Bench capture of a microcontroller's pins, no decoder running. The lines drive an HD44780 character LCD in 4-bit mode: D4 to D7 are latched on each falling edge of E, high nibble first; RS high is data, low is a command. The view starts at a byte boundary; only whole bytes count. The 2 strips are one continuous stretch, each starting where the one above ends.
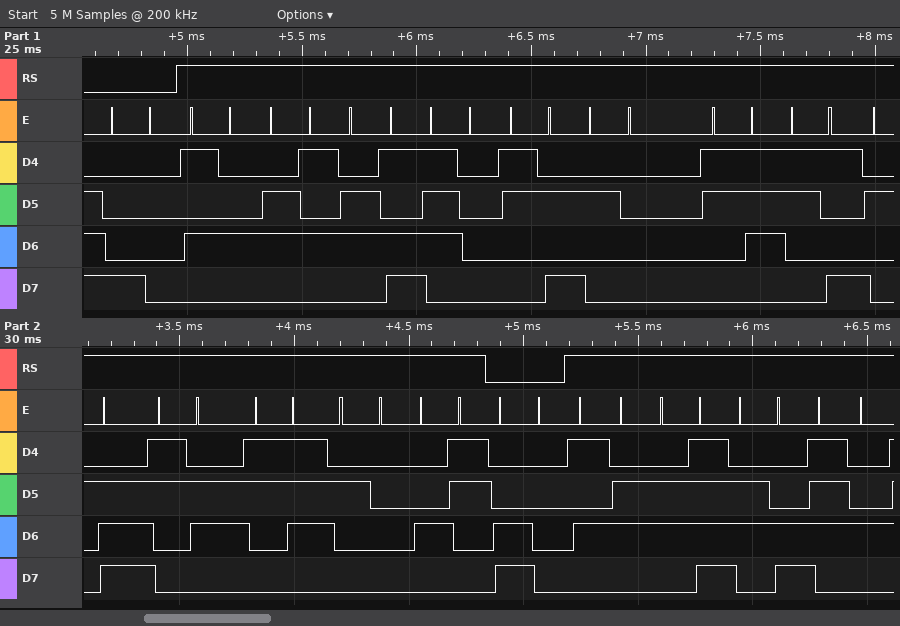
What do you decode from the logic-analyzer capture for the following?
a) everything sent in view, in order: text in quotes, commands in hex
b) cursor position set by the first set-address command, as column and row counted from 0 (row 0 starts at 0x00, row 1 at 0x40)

0x80 "Temp: 79.67 C" 0xC0 "Volt"
column 0, row 0
